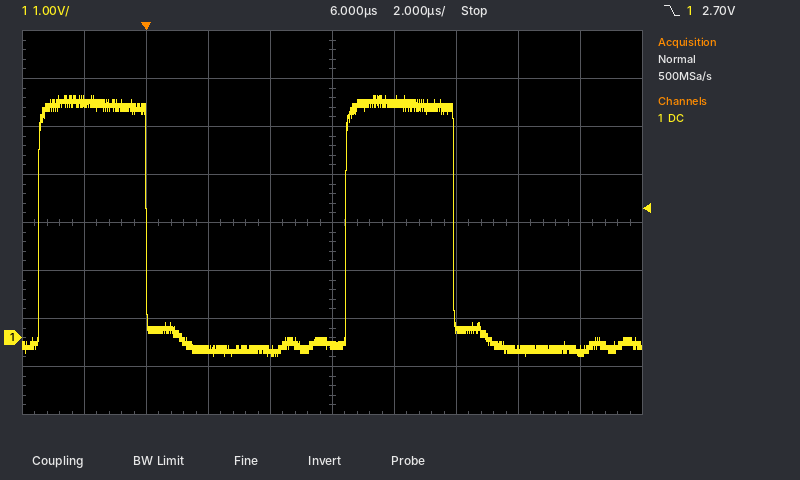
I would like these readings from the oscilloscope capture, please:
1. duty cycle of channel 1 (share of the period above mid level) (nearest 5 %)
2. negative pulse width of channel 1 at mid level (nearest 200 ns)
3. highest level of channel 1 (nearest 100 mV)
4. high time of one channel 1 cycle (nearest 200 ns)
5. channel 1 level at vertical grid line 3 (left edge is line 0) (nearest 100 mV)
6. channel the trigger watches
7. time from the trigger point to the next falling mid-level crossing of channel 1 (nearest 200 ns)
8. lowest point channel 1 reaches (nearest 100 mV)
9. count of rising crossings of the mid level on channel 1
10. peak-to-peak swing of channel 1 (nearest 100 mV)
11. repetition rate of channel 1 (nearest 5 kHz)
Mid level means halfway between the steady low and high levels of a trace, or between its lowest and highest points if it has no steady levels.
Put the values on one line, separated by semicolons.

35 %; 6.4 µs; 5.0 V; 3.4 µs; -200 mV; channel 1; 10.0 µs; -400 mV; 2; 5.4 V; 100 kHz
